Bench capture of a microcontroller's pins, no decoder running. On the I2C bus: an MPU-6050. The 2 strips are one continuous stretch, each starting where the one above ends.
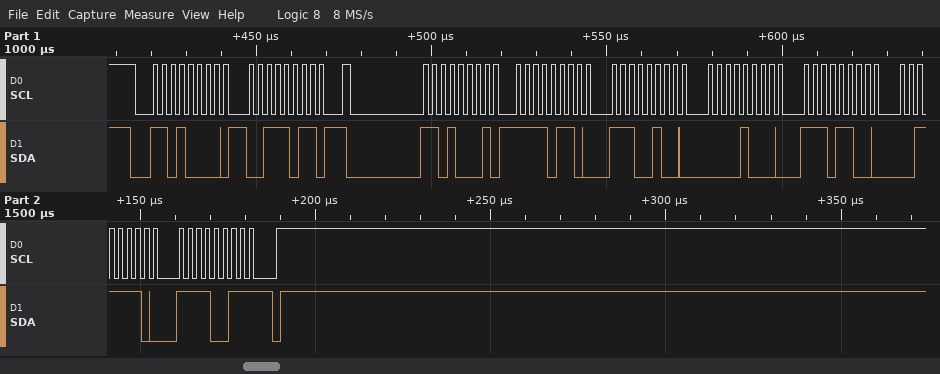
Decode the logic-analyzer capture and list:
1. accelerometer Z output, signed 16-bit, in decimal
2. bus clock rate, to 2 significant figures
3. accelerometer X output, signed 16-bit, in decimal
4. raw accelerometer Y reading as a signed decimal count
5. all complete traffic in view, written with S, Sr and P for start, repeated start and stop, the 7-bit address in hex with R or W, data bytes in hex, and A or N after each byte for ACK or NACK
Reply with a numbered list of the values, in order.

1. 16115
2. 400 kHz
3. -2332
4. 2284
5. S 68W A 3B A Sr 68R A F6 A E4 A 08 A EC A 3E A F3 N P
